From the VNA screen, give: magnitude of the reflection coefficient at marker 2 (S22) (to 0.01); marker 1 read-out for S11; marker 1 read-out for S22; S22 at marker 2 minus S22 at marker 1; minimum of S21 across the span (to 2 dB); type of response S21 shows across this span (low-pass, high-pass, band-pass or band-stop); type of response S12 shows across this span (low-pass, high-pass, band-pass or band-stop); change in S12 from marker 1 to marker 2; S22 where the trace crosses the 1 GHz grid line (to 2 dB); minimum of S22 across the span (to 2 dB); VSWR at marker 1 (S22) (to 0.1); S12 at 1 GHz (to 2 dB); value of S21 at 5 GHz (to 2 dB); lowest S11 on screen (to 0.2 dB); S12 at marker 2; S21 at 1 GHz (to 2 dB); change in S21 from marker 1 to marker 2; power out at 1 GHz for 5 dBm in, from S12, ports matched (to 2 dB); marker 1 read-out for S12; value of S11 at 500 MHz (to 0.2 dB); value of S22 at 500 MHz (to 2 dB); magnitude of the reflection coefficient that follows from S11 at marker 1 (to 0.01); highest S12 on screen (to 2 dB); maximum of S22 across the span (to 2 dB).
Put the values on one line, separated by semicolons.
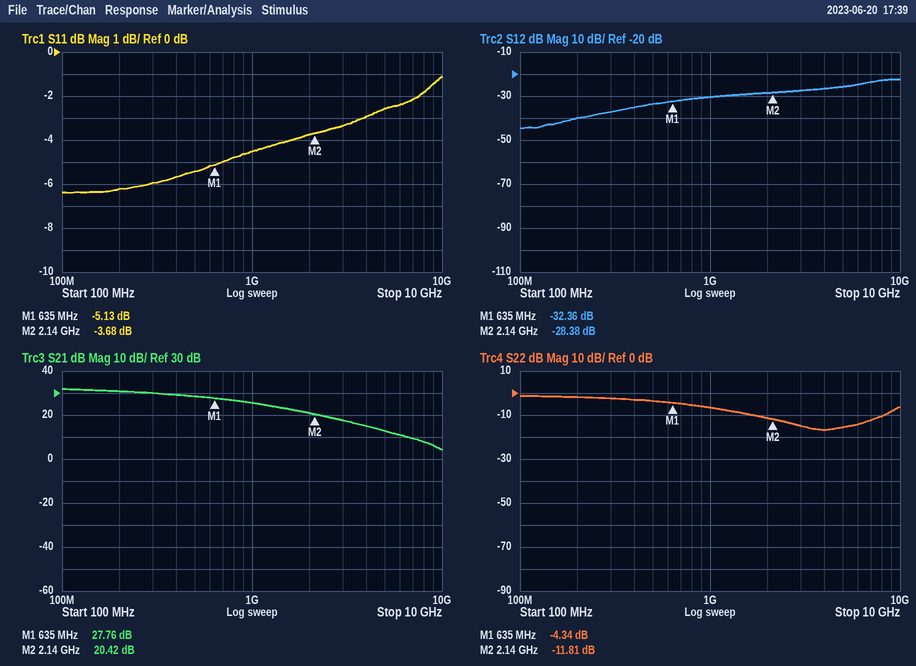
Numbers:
0.26; -5.13 dB; -4.34 dB; -7.47 dB; 4 dB; low-pass; high-pass; 3.98 dB; -6 dB; -16 dB; 4.1; -30 dB; 12 dB; -6.4 dB; -28.38 dB; 26 dB; -7.34 dB; -26 dBm; -32.36 dB; -5.4 dB; -4 dB; 0.55; -22 dB; -2 dB
